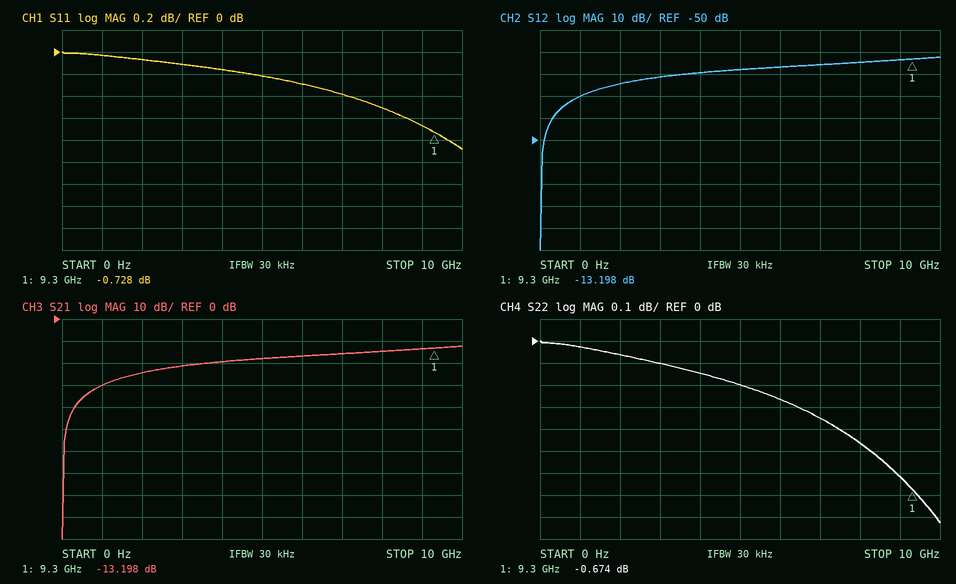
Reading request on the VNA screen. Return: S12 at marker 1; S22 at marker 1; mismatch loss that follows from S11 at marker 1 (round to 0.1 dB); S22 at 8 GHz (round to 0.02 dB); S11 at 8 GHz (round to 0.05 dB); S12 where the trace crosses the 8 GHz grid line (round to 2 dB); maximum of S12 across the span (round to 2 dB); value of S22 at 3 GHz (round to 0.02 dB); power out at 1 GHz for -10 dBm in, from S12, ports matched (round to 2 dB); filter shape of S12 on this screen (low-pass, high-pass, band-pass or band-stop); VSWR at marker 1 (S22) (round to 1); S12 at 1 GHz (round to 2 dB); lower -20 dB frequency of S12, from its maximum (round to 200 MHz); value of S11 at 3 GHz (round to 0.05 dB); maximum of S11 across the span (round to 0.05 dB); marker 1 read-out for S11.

-13.198 dB
-0.674 dB
8.1 dB
-0.46 dB
-0.50 dB
-14 dB
-12 dB
-0.10 dB
-40 dBm
high-pass
26
-30 dB
800 MHz
-0.10 dB
0.00 dB
-0.728 dB
